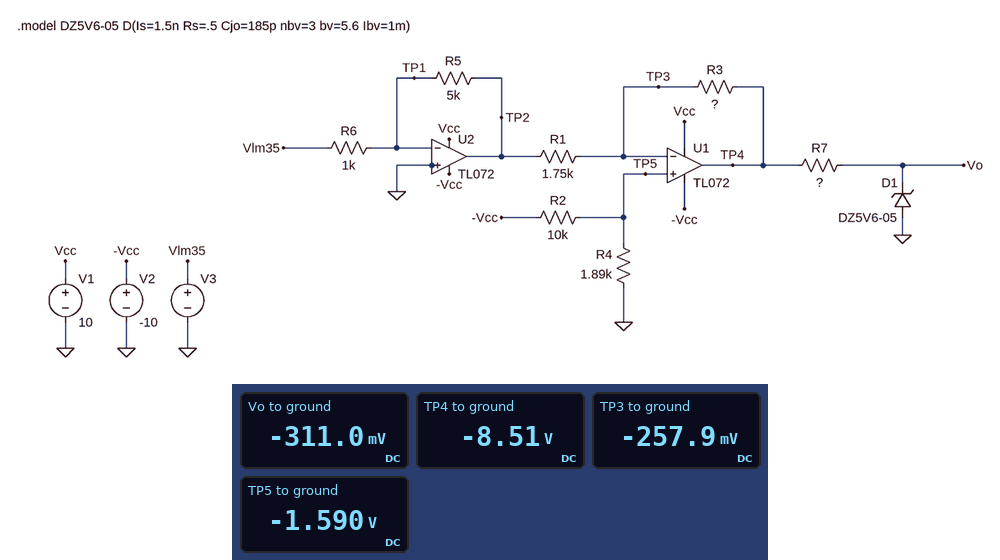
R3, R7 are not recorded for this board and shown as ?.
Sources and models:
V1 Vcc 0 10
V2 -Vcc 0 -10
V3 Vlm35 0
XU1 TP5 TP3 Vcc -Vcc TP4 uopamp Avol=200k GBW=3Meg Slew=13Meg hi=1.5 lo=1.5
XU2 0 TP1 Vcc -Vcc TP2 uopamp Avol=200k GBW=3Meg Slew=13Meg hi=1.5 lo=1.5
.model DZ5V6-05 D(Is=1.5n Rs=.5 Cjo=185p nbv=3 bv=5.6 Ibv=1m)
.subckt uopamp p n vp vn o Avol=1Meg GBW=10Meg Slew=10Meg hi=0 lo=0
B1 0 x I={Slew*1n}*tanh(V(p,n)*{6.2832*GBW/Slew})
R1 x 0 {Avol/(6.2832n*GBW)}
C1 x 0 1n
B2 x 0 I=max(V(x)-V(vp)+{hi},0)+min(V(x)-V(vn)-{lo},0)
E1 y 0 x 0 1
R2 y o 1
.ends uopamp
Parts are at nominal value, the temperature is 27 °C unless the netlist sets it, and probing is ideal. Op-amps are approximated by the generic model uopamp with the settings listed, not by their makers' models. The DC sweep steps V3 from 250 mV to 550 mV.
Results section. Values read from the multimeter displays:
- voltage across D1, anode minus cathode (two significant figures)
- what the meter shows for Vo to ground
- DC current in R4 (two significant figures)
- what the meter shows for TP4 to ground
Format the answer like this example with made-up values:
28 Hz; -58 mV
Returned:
310 mV; -311.0 mV; 840 µA; -8.51 V
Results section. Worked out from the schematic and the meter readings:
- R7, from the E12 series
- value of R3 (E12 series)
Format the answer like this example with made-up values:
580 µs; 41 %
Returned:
33 kΩ; 56 kΩ
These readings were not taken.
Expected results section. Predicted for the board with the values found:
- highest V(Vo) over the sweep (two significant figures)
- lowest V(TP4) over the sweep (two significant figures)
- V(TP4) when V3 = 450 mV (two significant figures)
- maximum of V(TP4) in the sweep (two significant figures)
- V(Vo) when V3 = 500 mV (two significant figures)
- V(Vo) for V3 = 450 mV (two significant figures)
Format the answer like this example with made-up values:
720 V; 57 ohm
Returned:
5.4 V; -8.5 V; 8.5 V; 8.5 V; 5.4 V; 5.4 V
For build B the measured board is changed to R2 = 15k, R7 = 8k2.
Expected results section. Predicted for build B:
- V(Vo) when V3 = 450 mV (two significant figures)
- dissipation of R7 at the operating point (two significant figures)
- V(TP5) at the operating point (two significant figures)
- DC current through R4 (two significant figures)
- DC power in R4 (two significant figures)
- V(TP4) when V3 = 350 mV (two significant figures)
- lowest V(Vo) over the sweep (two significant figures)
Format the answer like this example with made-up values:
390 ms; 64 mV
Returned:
5.5 V; 8.1 mW; -1.1 V; 590 µA; 660 µW; 8.5 V; 3.1 V
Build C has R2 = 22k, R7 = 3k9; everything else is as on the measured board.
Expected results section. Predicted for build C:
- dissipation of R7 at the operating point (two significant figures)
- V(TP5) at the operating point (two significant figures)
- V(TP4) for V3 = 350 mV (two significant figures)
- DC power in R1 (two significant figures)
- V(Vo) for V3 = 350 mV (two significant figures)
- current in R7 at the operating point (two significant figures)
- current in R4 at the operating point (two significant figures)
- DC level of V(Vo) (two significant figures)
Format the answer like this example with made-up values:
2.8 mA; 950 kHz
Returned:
17 mW; -790 mV; 8.5 V; 38 µW; 5.6 V; 2.1 mA; 420 µA; -370 mV
